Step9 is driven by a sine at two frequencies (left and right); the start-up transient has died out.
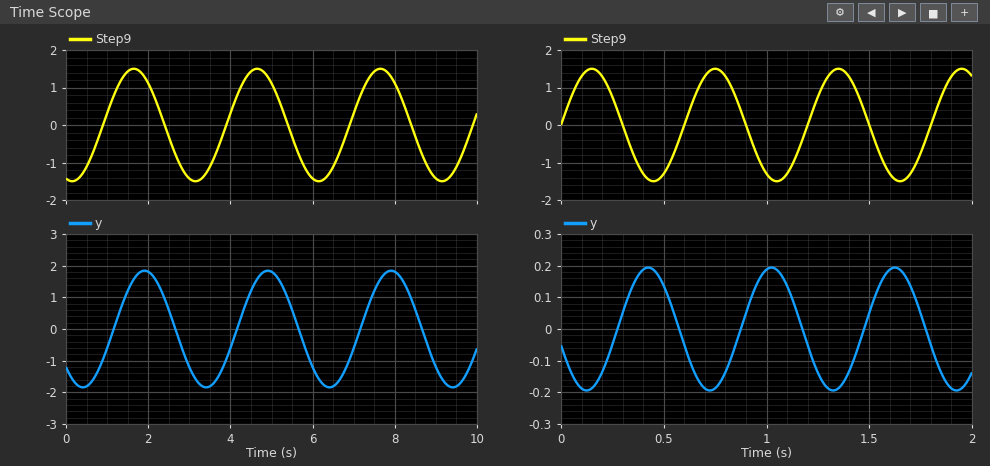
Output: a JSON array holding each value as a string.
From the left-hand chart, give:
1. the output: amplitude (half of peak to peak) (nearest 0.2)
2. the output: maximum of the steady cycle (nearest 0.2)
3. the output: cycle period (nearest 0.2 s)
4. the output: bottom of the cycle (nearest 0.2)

["1.8", "1.8", "3.0 s", "-1.8"]
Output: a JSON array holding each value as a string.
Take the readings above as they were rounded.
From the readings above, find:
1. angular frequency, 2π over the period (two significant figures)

["2.1 rad/s"]
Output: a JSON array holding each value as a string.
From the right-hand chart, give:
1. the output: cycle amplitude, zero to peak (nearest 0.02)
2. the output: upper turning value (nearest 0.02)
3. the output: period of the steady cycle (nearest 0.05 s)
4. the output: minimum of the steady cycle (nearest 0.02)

["0.20", "0.20", "0.60 s", "-0.20"]
